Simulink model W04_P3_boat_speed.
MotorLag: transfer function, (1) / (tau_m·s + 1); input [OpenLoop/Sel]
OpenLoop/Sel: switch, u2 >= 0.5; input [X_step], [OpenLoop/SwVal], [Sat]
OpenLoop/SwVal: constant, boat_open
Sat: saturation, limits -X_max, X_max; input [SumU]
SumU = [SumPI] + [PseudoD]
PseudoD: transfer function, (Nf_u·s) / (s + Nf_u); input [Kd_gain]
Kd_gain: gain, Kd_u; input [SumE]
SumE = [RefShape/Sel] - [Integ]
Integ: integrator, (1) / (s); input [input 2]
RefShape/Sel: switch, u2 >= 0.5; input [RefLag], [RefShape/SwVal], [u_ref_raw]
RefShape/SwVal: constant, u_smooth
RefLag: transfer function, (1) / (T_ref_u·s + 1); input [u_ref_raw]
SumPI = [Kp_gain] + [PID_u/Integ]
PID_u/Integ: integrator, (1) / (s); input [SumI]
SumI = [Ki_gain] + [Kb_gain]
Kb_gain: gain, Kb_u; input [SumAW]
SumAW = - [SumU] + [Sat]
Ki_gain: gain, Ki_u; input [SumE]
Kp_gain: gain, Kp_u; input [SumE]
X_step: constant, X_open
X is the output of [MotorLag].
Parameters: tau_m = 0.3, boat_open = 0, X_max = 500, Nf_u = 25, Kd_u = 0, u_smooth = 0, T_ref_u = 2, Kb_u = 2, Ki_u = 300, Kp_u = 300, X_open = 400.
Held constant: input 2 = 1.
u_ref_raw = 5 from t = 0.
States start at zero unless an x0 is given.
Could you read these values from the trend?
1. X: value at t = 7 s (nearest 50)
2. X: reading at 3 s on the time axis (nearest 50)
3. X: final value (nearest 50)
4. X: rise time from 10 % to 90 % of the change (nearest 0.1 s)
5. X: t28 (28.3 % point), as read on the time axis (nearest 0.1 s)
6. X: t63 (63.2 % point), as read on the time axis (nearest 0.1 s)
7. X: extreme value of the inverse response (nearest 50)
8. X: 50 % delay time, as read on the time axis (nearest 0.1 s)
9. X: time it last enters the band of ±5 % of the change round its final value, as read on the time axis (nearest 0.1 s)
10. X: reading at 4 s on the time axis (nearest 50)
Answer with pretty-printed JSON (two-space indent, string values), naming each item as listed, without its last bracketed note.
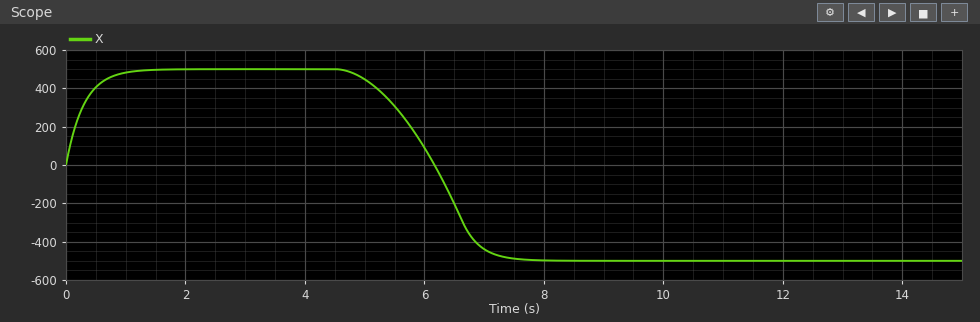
{
  "X: value at t = 7 s": "-450",
  "X: reading at 3 s on the time axis": "500",
  "X: final value": "-500",
  "X: rise time from 10 % to 90 % of the change": "0.8 s",
  "X: t28 (28.3 % point), as read on the time axis": "6.4 s",
  "X: t63 (63.2 % point), as read on the time axis": "6.7 s",
  "X: extreme value of the inverse response": "500",
  "X: 50 % delay time, as read on the time axis": "6.6 s",
  "X: time it last enters the band of ±5 % of the change round its final value, as read on the time axis": "7.3 s",
  "X: reading at 4 s on the time axis": "500"
}
